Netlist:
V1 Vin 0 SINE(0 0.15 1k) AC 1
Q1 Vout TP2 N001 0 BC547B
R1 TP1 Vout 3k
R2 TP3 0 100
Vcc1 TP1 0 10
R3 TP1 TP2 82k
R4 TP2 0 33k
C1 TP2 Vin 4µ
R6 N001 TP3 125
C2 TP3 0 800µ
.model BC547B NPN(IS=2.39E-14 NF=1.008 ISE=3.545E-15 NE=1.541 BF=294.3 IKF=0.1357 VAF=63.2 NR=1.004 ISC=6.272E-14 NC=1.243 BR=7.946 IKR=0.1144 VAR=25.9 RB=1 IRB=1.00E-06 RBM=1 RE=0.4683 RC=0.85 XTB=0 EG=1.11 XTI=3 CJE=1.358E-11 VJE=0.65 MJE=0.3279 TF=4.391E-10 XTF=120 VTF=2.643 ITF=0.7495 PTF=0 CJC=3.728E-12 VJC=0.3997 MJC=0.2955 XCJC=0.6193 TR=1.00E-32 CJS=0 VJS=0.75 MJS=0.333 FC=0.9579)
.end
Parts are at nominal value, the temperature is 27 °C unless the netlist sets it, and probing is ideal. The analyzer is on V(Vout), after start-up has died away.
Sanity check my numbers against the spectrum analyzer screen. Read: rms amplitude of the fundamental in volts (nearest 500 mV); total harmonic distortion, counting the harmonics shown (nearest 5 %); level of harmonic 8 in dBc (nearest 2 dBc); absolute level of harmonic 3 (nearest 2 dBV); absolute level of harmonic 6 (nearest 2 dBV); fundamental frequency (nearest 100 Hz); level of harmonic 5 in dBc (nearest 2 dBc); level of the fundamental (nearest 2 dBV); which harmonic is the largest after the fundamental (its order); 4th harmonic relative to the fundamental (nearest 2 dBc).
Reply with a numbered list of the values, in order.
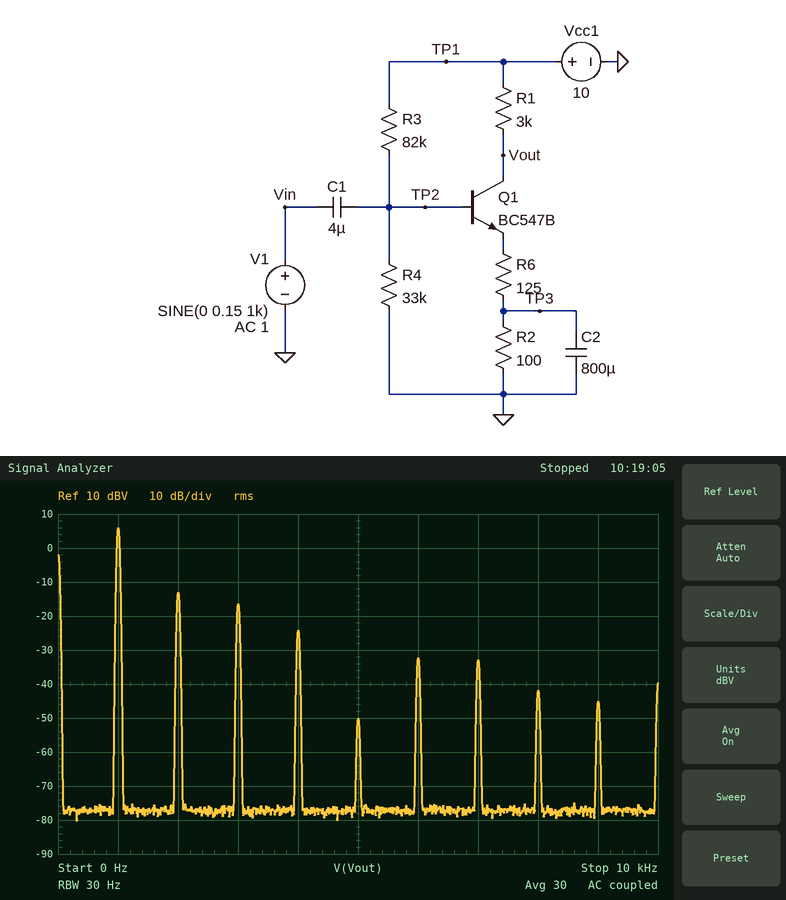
1. 2.0 V
2. 15 %
3. -48 dBc
4. -16 dBV
5. -32 dBV
6. 1.0 kHz
7. -56 dBc
8. 6 dBV
9. 2
10. -30 dBc
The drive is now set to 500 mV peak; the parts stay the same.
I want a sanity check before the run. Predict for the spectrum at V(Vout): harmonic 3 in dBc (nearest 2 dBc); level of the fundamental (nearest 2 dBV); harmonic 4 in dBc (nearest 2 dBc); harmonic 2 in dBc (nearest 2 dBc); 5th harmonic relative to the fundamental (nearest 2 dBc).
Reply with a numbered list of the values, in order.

1. -20 dBc
2. 12 dBV
3. -18 dBc
4. -10 dBc
5. -36 dBc
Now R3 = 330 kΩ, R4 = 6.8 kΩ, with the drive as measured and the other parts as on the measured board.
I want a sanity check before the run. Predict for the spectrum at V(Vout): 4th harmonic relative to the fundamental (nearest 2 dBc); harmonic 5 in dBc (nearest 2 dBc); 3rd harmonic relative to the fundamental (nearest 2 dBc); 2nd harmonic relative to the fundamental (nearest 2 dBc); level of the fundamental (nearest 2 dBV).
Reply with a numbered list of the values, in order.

1. -12 dBc
2. -18 dBc
3. -6 dBc
4. -2 dBc
5. -98 dBV
